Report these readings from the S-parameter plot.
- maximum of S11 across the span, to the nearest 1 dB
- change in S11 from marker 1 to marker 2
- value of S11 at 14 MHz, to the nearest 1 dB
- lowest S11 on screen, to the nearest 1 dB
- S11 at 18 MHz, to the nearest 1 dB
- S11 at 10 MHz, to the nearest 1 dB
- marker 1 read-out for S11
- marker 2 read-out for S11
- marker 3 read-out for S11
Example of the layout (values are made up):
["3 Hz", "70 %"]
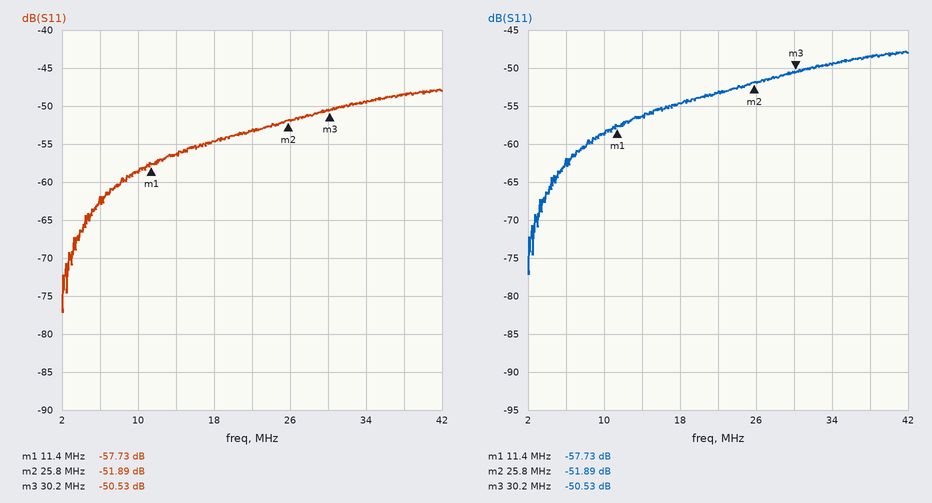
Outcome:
["-48 dB", "5.84 dB", "-56 dB", "-77 dB", "-55 dB", "-59 dB", "-57.73 dB", "-51.89 dB", "-50.53 dB"]
